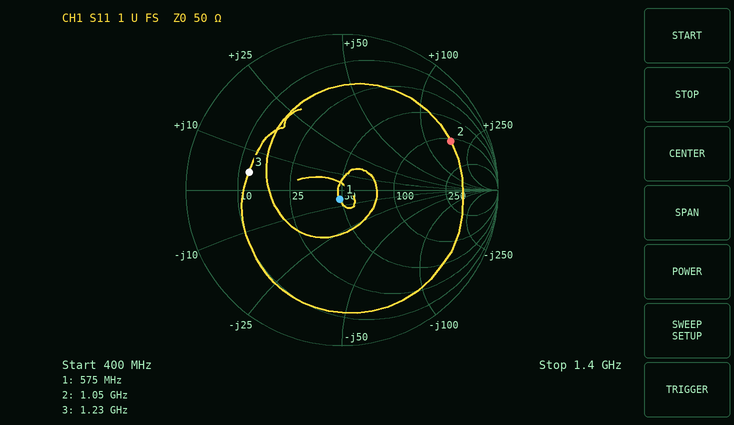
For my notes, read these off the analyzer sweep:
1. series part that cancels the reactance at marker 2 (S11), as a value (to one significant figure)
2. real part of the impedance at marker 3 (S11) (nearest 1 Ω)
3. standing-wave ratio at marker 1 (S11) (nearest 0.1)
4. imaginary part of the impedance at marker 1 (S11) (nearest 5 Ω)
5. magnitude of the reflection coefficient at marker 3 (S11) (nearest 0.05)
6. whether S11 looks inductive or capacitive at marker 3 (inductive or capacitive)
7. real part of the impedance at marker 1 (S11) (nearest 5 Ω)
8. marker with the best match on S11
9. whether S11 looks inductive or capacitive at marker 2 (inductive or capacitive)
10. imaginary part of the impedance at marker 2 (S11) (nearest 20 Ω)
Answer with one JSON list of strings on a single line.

["900 fF", "12 Ω", "1.1", "-5 Ω", "0.60", "inductive", "50 Ω", "marker 1", "inductive", "+160 Ω"]
